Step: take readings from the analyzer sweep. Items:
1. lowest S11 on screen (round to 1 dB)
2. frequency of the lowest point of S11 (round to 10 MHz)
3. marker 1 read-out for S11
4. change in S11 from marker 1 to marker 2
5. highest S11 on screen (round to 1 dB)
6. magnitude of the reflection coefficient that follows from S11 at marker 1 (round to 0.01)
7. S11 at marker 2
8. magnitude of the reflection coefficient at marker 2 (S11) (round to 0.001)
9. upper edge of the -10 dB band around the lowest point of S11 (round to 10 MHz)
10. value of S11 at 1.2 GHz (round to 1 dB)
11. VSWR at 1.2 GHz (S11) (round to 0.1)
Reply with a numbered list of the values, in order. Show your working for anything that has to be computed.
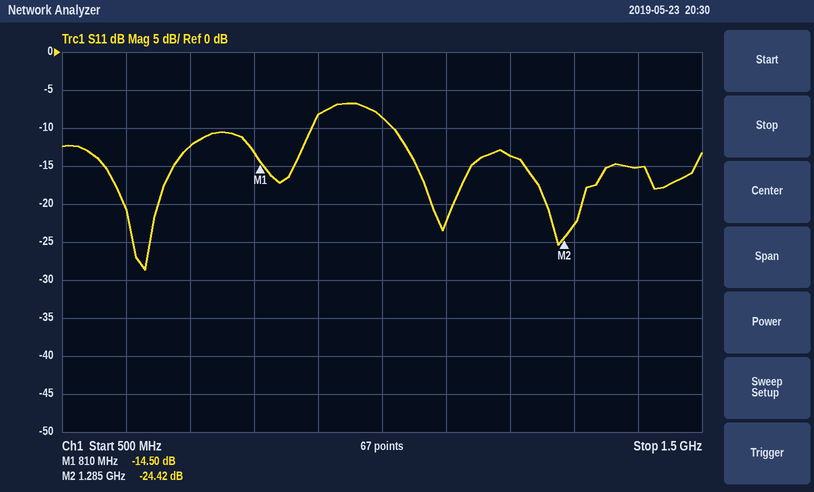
1. -29 dB
2. 630 MHz
3. -14.50 dB
4. -24.42 − (-14.5) = -9.92 dB
5. -7 dB
6. 10^(-14.5/20) ≈ 0.19
7. -24.42 dB
8. 10^(-24.42/20) ≈ 0.060
9. 890 MHz
10. -14 dB
11. |Γ| = 10^(-14/20) = 0.1995; VSWR = (1 + 0.1995)/(1 − 0.1995) ≈ 1.5
